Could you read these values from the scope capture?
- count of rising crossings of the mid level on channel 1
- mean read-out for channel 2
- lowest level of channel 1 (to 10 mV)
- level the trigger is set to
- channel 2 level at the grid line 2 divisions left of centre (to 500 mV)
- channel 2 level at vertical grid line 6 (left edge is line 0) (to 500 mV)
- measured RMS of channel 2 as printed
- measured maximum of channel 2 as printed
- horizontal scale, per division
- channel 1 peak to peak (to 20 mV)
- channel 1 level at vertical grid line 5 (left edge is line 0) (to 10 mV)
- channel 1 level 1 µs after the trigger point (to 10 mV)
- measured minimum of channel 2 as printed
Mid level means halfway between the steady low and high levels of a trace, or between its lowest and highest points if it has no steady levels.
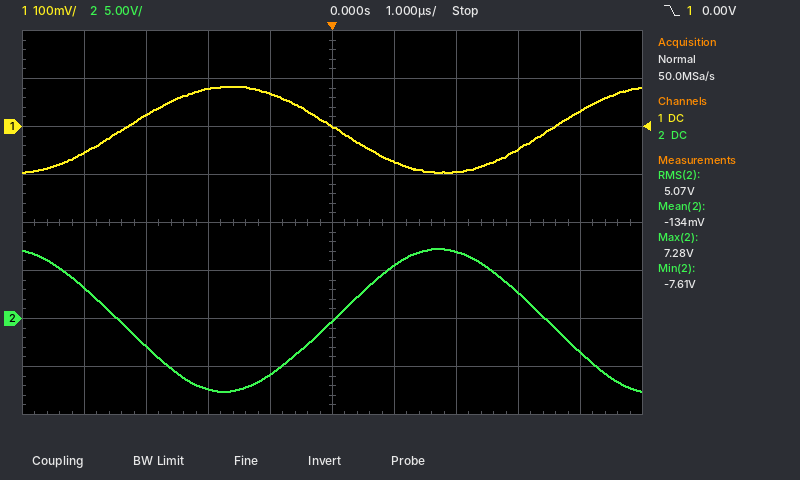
2
-134 mV
-100 mV
0.00 V
-7.5 V
5.5 V
5.07 V
7.28 V
1 µs
180 mV
0 mV
-70 mV
-7.61 V
